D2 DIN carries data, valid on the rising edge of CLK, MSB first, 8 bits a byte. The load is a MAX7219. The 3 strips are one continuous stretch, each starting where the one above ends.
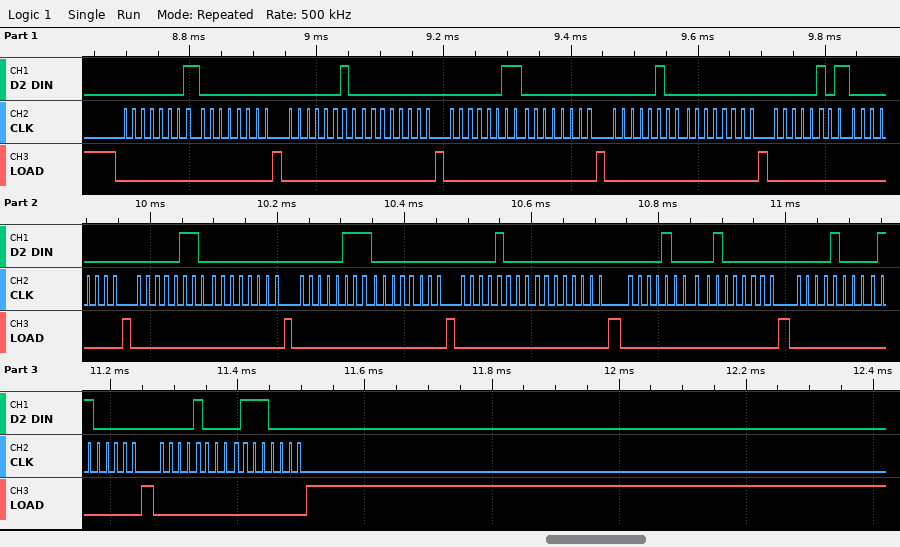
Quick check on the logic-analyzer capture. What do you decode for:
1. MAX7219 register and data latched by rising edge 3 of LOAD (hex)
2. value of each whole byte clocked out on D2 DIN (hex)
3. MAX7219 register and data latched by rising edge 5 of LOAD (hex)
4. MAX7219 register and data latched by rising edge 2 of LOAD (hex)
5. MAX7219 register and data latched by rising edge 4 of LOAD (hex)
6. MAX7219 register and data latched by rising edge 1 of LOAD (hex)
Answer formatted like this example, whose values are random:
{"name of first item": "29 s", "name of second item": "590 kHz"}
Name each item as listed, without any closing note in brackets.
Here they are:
{"MAX7219 register and data latched by rising edge 3 of LOAD": "register 0x3, data 0x00", "value of each whole byte clocked out on D2 DIN": "01 00 02 00 03 00 04 00 05 00 06 00 07 00 08 00 08 40 08 60 08 70", "MAX7219 register and data latched by rising edge 5 of LOAD": "register 0x5, data 0x00", "MAX7219 register and data latched by rising edge 2 of LOAD": "register 0x2, data 0x00", "MAX7219 register and data latched by rising edge 4 of LOAD": "register 0x4, data 0x00", "MAX7219 register and data latched by rising edge 1 of LOAD": "register 0x1, data 0x00"}
